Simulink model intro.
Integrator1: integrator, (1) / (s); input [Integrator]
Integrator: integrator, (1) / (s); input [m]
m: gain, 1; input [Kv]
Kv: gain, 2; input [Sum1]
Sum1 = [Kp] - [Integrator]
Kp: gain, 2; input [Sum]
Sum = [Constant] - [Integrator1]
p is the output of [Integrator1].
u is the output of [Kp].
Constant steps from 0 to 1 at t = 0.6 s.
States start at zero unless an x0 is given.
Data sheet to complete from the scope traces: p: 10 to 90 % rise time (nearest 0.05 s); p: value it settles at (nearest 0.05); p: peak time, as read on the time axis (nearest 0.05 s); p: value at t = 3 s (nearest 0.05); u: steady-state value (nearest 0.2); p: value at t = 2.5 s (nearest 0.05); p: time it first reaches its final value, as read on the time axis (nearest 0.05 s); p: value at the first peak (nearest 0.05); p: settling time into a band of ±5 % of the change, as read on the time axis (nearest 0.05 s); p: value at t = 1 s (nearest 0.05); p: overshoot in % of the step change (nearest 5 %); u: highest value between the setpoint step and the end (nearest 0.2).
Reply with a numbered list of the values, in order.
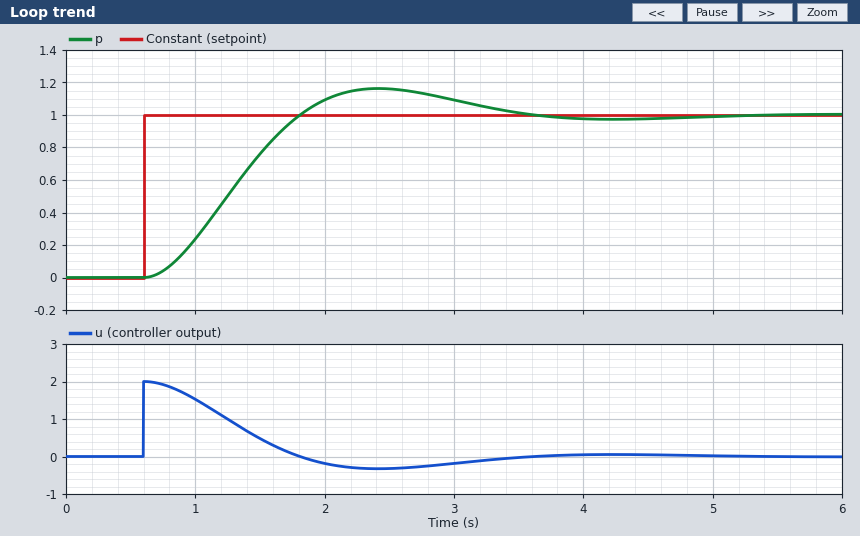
1. 0.80 s
2. 1.00
3. 2.40 s
4. 1.10
5. 0.0
6. 1.15
7. 1.80 s
8. 1.15
9. 3.25 s
10. 0.25
11. 15 %
12. 2.0
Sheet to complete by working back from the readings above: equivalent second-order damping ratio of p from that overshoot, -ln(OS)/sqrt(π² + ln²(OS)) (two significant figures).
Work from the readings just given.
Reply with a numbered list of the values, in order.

1. 0.52
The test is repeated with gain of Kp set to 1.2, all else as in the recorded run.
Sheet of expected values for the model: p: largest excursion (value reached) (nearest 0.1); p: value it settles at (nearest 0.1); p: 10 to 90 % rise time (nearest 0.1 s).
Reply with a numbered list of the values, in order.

1. 1.1
2. 1.0
3. 1.3 s
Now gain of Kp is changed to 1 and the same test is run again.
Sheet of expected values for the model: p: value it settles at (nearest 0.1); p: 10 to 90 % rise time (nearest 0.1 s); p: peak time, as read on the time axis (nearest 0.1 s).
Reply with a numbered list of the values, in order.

1. 1.0
2. 1.5 s
3. 3.7 s
